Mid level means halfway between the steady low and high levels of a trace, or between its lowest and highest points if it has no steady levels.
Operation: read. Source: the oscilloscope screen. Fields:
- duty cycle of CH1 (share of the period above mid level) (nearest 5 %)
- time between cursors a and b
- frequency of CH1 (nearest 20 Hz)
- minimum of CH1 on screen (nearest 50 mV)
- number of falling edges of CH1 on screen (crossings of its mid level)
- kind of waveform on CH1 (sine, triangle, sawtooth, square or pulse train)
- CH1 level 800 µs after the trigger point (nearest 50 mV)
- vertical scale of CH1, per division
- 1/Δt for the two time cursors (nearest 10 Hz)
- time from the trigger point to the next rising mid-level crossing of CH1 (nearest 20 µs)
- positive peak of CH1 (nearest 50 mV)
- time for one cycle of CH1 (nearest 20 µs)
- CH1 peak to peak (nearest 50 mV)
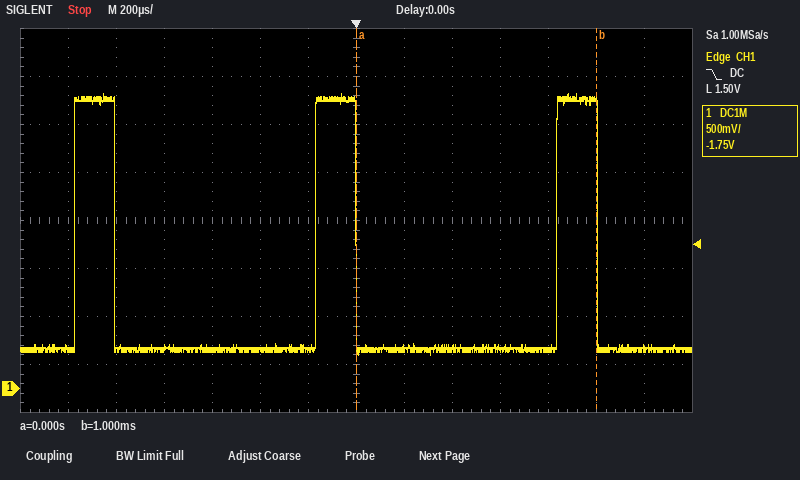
15 %
1.00 ms
1.00 kHz
350 mV
3
pulse train
400 mV
500 mV
1.00 kHz
840 µs
3.05 V
1.00 ms
2.70 V
